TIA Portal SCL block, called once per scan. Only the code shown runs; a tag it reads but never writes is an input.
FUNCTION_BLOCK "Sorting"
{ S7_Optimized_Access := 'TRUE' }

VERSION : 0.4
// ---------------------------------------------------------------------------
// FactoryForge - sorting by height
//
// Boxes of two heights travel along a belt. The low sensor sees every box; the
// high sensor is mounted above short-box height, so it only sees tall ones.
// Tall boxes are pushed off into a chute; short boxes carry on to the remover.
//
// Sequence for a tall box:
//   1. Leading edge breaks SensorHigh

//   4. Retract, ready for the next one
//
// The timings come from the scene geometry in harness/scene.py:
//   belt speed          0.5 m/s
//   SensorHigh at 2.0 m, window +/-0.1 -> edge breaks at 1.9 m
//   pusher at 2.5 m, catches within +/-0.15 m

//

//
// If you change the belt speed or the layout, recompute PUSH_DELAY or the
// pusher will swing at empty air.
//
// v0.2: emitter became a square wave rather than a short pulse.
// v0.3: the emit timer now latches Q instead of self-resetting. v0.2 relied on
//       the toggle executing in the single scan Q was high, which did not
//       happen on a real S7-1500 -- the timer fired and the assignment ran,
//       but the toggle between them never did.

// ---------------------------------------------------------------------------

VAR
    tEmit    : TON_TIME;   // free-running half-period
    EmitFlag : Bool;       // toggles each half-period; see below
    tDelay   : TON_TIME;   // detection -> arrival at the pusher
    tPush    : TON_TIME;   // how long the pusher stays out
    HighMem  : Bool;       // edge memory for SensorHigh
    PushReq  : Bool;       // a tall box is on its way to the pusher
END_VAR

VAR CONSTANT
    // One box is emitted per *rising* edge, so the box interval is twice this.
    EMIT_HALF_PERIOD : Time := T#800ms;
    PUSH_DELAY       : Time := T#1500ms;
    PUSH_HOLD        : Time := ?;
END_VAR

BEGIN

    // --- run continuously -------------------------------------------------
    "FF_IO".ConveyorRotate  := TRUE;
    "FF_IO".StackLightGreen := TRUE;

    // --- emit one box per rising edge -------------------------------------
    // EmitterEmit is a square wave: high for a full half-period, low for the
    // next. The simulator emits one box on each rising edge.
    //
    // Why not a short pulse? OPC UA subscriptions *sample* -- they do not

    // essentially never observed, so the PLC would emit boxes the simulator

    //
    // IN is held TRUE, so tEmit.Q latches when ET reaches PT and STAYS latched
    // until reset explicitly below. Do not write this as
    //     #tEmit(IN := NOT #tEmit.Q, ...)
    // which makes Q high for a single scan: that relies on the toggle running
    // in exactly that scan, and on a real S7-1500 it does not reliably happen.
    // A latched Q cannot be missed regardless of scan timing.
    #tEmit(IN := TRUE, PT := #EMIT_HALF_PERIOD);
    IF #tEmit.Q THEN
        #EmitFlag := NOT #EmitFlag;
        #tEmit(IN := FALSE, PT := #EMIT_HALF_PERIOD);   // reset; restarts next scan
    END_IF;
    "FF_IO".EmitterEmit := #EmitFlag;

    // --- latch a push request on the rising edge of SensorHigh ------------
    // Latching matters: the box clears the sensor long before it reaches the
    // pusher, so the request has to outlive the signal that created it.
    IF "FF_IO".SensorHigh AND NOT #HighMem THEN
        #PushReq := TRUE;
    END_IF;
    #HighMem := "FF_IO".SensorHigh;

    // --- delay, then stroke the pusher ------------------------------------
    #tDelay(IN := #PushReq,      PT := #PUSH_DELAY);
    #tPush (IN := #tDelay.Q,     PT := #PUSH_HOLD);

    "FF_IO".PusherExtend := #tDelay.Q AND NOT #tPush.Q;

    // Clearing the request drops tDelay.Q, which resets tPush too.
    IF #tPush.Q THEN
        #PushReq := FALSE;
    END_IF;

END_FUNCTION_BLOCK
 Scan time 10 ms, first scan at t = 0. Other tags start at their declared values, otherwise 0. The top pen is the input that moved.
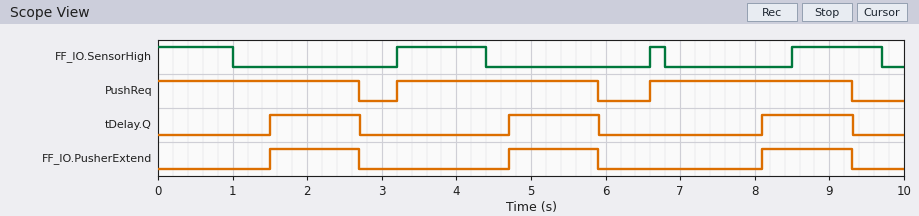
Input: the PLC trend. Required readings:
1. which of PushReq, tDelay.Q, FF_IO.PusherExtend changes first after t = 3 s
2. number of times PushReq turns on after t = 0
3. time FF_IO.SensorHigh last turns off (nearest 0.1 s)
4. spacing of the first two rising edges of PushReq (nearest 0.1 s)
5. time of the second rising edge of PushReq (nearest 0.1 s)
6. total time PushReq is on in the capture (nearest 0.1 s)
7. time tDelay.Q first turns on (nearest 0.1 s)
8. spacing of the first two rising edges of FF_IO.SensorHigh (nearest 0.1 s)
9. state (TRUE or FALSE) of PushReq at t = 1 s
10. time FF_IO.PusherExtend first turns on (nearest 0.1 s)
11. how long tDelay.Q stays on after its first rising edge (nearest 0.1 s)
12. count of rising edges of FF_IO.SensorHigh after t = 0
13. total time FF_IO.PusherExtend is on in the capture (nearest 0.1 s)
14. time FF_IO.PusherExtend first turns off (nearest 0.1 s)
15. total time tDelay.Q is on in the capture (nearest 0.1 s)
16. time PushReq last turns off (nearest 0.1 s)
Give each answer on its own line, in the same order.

PushReq
2
9.7 s
3.4 s
6.6 s
8.1 s
1.5 s
3.4 s
TRUE
1.5 s
1.2 s
3
3.6 s
2.7 s
3.6 s
9.3 s
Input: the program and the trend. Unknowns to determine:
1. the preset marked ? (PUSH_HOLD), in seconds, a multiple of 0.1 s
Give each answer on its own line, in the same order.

1.2 s
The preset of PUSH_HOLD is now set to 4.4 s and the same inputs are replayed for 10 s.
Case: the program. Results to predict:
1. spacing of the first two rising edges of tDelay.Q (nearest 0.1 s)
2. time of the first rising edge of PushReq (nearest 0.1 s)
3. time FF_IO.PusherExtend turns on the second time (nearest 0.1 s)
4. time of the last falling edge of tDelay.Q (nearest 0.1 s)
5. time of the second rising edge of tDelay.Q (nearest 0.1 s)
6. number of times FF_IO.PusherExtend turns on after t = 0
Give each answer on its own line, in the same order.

6.6 s
6.6 s
8.1 s
5.9 s
8.1 s
2
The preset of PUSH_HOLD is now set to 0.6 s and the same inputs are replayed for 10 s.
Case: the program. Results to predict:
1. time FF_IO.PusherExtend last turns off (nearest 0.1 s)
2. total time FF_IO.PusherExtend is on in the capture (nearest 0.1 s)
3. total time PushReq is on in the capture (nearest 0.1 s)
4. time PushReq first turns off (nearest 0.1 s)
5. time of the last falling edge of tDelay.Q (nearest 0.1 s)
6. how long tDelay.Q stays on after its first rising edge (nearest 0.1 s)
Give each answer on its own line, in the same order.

8.7 s
1.8 s
6.3 s
2.1 s
8.7 s
0.6 s
